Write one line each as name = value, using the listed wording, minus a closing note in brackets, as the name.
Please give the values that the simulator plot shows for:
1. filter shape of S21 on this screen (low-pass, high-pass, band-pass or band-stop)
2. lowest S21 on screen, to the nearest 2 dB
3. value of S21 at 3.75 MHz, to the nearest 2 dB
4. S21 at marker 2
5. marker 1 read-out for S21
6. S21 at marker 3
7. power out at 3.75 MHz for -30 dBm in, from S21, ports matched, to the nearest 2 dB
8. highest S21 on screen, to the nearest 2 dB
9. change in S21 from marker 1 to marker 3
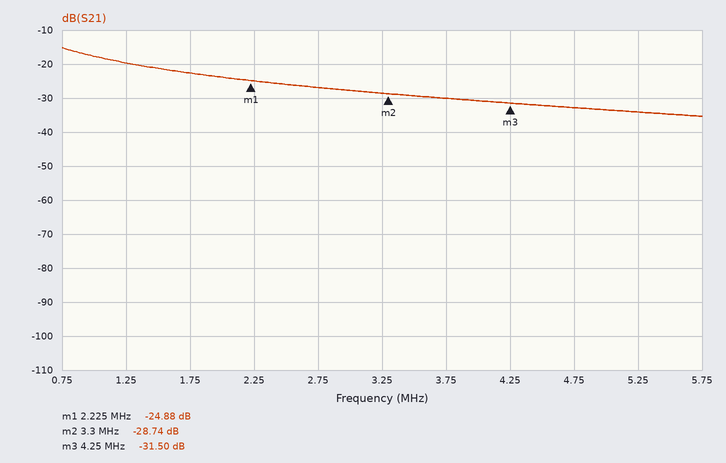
filter shape of S21 on this screen = low-pass
lowest S21 on screen, to the nearest 2 dB = -36 dB
value of S21 at 3.75 MHz, to the nearest 2 dB = -30 dB
S21 at marker 2 = -28.74 dB
marker 1 read-out for S21 = -24.88 dB
S21 at marker 3 = -31.50 dB
power out at 3.75 MHz for -30 dBm in, from S21, ports matched, to the nearest 2 dB = -60 dBm
highest S21 on screen, to the nearest 2 dB = -16 dB
change in S21 from marker 1 to marker 3 = -6.62 dB
